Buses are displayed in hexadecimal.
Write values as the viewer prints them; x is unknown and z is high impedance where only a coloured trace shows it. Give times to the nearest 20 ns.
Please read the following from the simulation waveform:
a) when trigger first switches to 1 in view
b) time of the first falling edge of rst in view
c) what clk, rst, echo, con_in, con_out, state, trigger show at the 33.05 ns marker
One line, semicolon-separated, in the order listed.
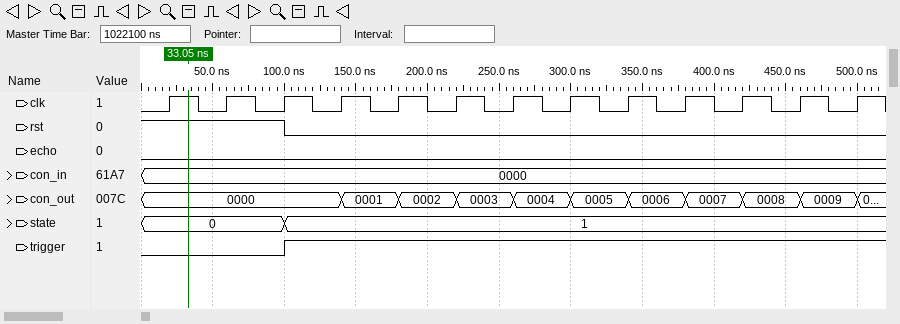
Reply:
100 ns; 100 ns; clk=1, rst=1, echo=0, con_in=0000, con_out=0000, state=0, trigger=0
